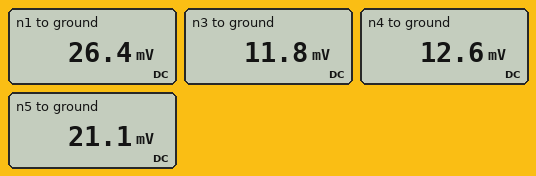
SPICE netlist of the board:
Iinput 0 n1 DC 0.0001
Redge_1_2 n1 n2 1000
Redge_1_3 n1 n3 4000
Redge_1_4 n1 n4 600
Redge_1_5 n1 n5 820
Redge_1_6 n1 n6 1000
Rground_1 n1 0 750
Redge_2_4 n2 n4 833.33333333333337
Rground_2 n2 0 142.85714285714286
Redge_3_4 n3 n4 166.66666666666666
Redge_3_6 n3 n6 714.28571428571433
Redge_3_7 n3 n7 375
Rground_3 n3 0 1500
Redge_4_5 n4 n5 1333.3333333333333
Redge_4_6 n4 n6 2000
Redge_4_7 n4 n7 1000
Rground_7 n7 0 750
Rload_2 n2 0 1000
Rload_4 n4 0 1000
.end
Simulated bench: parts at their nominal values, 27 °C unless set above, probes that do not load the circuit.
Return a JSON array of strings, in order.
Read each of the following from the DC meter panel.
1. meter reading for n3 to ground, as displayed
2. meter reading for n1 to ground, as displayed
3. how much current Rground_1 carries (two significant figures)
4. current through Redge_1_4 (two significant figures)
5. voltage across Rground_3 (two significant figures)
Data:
["11.8 mV", "26.4 mV", "35 µA", "23 µA", "12 mV"]
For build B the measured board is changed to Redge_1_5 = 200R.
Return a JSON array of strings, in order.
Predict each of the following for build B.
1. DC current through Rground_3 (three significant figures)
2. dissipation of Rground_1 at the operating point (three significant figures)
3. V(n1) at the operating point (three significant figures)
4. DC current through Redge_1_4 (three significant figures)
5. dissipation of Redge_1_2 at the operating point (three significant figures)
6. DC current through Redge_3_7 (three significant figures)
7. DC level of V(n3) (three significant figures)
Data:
["7.96 µA", "905 nW", "26.1 mV", "22.0 µA", "484 nW", "8.01 µA", "11.9 mV"]
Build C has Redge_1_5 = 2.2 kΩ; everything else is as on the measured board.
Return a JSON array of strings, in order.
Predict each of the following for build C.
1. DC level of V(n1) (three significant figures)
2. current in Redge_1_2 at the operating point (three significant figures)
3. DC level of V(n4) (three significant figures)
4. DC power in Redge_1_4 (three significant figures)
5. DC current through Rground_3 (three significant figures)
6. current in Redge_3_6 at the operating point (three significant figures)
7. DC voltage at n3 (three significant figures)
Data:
["26.8 mV", "22.7 µA", "12.4 mV", "345 nW", "7.76 µA", "7.48 µA", "11.6 mV"]
